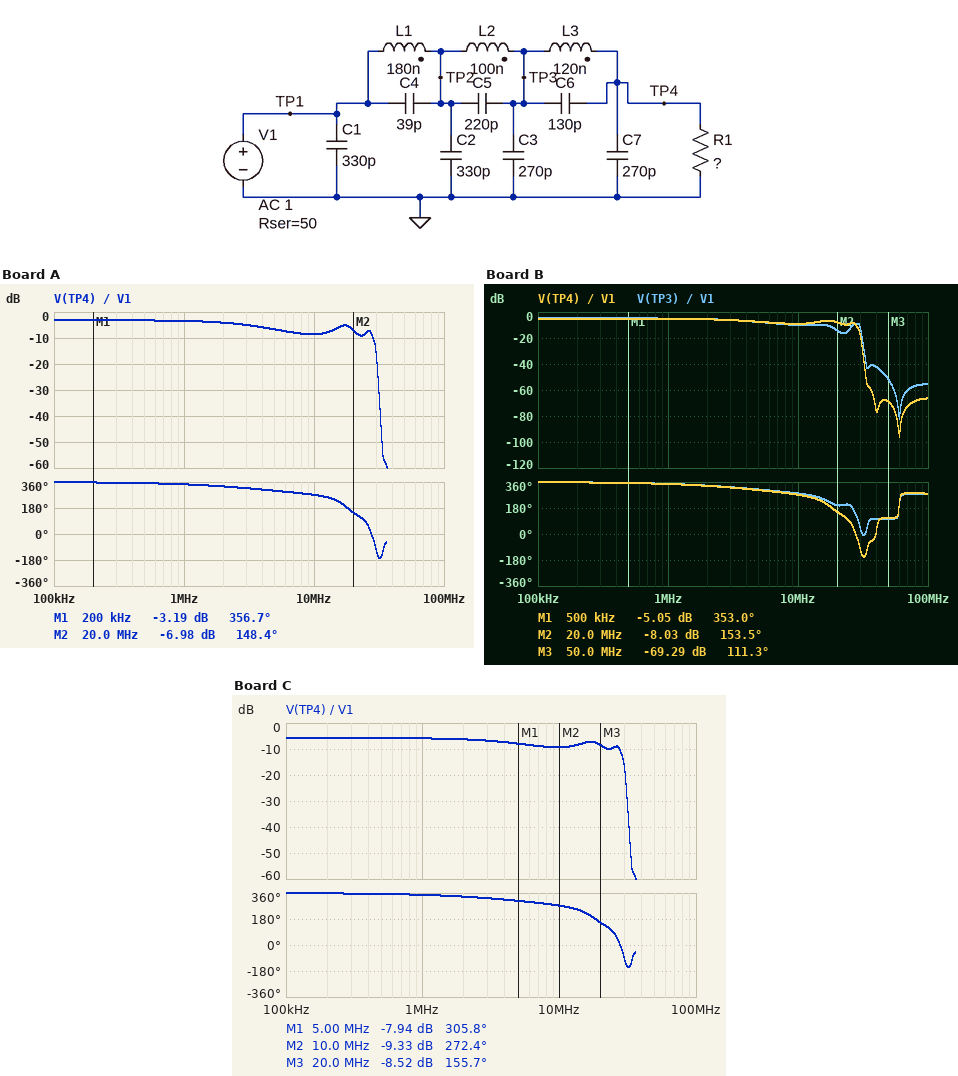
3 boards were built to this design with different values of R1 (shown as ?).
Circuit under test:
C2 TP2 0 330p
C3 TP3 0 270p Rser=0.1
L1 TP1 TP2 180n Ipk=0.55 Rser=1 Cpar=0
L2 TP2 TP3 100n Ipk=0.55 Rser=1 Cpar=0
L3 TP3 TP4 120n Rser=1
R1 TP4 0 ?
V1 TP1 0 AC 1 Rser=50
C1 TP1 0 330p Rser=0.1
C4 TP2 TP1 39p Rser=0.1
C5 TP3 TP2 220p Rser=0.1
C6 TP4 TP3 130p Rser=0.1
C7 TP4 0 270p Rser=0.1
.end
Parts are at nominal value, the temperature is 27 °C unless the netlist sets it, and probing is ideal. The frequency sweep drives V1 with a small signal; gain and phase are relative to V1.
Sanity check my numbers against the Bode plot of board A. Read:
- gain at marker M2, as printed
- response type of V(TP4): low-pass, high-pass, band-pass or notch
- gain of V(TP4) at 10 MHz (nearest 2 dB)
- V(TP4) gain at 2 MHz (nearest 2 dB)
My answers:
-6.98 dB
low-pass
-8 dB
-4 dB
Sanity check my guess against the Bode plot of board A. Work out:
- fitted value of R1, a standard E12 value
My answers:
120 Ω
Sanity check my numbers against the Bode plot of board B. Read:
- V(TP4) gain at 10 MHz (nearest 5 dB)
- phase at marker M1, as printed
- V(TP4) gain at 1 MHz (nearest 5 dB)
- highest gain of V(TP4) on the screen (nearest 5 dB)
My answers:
-10 dB
353.0 deg
-5 dB
-5 dB
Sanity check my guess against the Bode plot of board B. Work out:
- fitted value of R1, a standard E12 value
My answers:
68 Ω
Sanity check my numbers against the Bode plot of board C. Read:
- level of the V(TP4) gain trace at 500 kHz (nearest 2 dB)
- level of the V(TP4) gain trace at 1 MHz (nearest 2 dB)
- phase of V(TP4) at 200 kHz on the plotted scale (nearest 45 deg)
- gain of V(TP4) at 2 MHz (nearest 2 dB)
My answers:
-6 dB
-6 dB
360 deg
-6 dB
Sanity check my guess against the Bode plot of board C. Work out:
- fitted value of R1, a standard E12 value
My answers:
56 Ω
